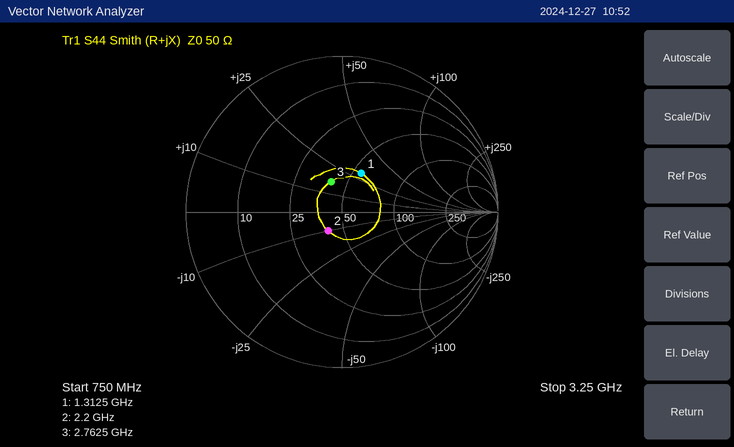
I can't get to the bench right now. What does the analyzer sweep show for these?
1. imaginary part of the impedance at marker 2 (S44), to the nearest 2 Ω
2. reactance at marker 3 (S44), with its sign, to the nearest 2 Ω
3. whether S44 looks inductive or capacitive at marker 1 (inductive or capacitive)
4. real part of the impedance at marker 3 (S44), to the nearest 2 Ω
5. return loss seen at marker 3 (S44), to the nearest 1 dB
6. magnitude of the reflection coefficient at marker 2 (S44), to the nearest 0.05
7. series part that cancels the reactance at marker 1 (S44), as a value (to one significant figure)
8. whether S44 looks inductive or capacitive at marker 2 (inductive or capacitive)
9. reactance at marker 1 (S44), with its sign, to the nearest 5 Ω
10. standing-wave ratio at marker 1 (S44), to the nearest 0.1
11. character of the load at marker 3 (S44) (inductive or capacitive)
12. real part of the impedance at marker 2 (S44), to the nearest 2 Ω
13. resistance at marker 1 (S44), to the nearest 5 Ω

-10 Ω
+16 Ω
inductive
40 Ω
14 dB
0.15
4 pF
capacitive
+30 Ω
1.8
inductive
40 Ω
55 Ω
